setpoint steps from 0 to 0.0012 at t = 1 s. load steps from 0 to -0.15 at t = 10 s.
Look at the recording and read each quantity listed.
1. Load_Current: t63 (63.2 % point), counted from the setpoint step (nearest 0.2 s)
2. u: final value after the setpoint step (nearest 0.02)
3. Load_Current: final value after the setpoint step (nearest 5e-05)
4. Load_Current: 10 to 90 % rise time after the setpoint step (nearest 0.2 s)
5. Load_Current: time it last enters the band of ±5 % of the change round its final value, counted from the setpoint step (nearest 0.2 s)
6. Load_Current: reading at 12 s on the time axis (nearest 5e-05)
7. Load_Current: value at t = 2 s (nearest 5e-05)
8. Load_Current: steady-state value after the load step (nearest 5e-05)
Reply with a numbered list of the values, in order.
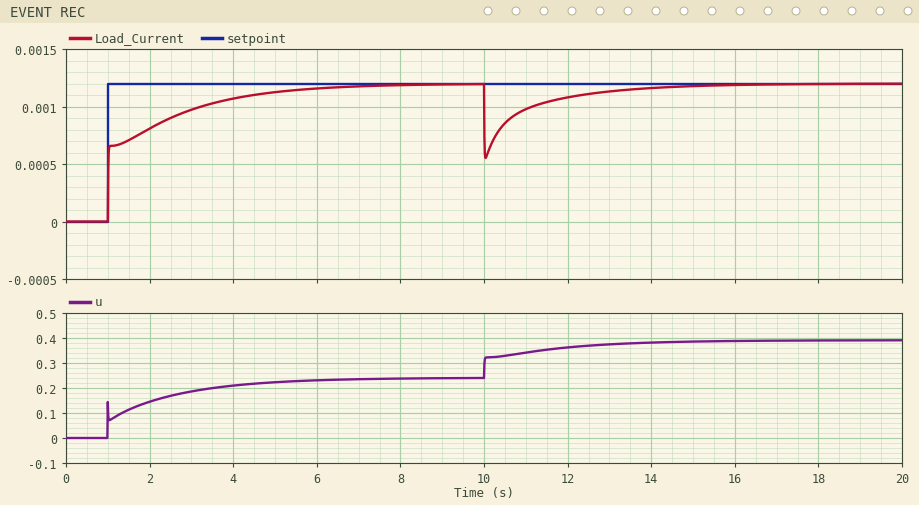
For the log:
1. 0.8 s
2. 0.24
3. 0.00120
4. 3.2 s
5. 4.4 s
6. 0.00110
7. 0.00080
8. 0.00120
